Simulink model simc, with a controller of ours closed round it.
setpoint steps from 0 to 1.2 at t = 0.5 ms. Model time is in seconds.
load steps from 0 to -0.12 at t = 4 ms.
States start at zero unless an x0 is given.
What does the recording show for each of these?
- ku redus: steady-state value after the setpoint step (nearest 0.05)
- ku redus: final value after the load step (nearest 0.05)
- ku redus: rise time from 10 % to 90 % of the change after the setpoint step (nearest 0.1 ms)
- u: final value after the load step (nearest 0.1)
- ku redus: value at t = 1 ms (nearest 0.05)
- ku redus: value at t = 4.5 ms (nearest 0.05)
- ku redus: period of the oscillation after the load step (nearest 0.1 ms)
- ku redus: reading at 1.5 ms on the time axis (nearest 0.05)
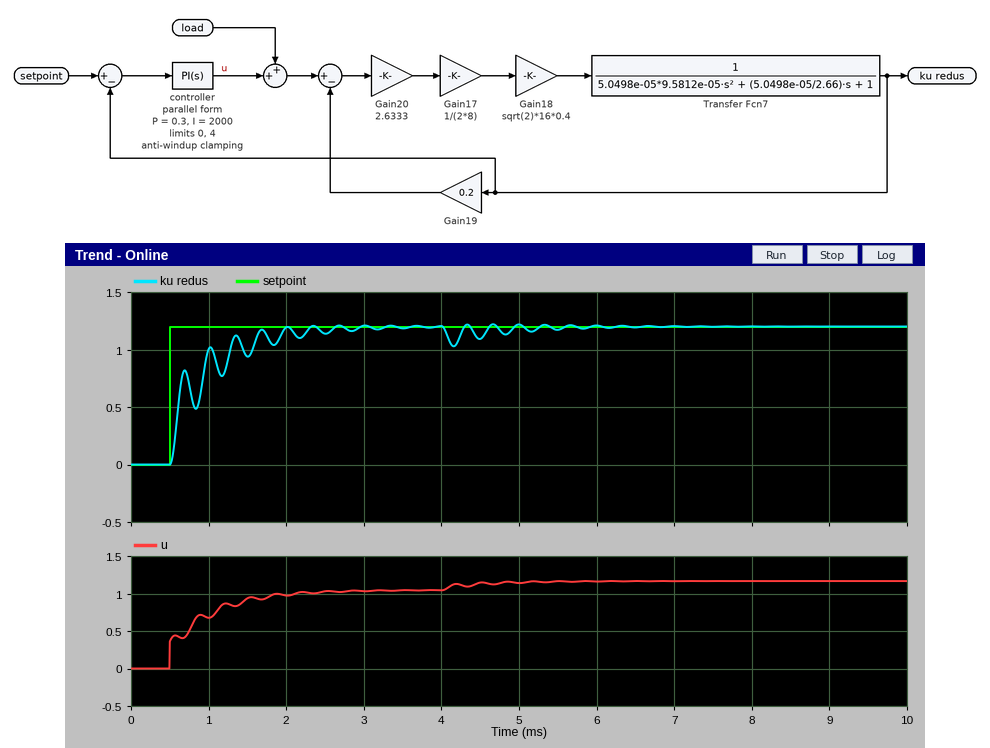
1.20
1.20
0.8 ms
1.2
1.00
1.10
0.3 ms
0.95
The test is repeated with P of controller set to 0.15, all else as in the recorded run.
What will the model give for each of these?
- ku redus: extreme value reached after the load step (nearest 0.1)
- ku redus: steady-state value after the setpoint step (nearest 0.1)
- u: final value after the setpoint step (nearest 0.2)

1.0
1.2
1.0
